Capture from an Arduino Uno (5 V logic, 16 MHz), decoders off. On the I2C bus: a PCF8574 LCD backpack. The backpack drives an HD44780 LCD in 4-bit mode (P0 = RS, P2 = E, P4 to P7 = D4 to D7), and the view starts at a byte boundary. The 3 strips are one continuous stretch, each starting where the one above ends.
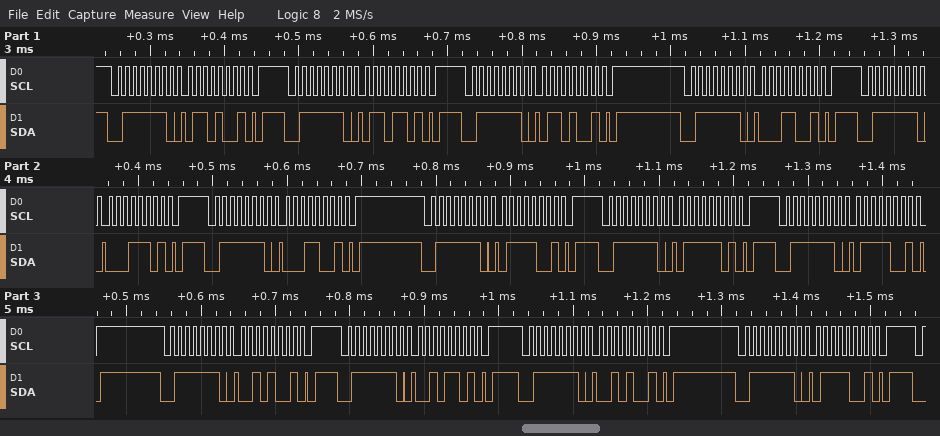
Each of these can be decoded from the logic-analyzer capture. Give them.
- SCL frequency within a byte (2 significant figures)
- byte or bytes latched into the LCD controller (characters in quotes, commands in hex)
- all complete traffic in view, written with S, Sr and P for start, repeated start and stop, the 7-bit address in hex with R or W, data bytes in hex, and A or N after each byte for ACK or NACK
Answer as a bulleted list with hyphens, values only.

- 100 kHz
- 'a' 'r'
- S 3FW A 69 A P S 3FW A 6D A P S 3FW A 69 A P S 3FW A 19 A P S 3FW A 1D A P S 3FW A 19 A P S 3FW A 79 A P S 3FW A 7D A P S 3FW A 79 A P S 3FW A 29 A P S 3FW A 2D A P S 3FW A 29 A P S 3FW A 79 A P
